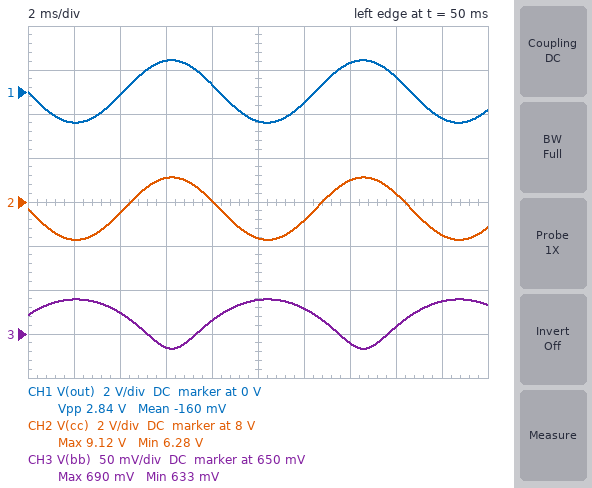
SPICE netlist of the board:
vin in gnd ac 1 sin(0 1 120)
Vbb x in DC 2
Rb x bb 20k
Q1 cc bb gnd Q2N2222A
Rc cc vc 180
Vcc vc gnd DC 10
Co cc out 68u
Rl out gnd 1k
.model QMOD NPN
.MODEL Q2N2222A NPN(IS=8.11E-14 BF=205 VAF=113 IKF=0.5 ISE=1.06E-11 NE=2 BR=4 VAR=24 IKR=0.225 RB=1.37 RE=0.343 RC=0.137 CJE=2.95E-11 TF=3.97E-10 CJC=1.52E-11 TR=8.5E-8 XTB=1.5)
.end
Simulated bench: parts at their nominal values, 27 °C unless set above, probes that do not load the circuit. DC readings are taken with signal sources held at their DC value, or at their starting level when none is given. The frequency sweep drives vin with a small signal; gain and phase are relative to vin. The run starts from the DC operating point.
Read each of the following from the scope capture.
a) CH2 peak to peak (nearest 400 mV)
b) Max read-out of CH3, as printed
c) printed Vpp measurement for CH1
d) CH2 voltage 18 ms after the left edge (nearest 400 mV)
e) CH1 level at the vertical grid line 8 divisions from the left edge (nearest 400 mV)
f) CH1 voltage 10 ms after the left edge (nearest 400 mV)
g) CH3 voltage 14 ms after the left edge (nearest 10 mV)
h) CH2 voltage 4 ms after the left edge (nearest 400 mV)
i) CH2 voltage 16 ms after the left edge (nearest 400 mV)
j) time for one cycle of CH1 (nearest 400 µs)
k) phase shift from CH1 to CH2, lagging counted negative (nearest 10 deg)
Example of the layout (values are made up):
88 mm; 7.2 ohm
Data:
2.8 V; 690 mV; 2.84 V; 6.4 V; 800 mV; -1.2 V; 640 mV; 7.6 V; 8.4 V; 8.4 ms; 0 deg
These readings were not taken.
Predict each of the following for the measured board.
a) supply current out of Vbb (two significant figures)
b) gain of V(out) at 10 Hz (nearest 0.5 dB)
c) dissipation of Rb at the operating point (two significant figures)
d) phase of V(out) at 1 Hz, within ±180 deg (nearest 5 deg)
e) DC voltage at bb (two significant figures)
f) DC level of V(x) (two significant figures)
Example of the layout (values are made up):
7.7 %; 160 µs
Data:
66 µA; 3.0 dB; 88 µW; -115 deg; 670 mV; 2.0 V
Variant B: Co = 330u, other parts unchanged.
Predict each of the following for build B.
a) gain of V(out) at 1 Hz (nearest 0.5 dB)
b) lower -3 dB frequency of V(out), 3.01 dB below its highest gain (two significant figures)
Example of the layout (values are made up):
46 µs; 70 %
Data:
2.5 dB; 410 mHz
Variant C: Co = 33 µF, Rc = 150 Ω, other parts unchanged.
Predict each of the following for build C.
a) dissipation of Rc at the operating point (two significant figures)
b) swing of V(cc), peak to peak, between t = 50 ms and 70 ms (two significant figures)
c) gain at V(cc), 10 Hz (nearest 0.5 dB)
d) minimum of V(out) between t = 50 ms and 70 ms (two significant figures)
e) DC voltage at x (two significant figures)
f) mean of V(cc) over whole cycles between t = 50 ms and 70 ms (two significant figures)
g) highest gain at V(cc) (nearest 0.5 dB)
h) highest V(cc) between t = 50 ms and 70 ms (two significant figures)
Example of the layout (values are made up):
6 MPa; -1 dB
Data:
25 mW; 2.4 V; 2.0 dB; -1.2 V; 2.0 V; 8.1 V; 3.0 dB; 9.3 V
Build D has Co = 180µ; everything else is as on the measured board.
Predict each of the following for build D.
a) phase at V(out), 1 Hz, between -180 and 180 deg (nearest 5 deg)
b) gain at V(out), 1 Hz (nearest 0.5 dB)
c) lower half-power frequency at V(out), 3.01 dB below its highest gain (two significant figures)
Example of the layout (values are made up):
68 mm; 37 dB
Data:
-145 deg; 1.0 dB; 750 mHz
